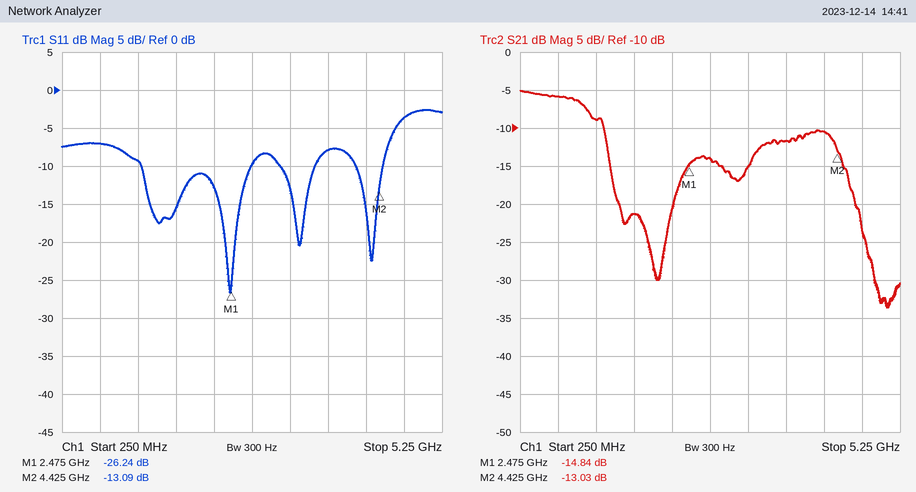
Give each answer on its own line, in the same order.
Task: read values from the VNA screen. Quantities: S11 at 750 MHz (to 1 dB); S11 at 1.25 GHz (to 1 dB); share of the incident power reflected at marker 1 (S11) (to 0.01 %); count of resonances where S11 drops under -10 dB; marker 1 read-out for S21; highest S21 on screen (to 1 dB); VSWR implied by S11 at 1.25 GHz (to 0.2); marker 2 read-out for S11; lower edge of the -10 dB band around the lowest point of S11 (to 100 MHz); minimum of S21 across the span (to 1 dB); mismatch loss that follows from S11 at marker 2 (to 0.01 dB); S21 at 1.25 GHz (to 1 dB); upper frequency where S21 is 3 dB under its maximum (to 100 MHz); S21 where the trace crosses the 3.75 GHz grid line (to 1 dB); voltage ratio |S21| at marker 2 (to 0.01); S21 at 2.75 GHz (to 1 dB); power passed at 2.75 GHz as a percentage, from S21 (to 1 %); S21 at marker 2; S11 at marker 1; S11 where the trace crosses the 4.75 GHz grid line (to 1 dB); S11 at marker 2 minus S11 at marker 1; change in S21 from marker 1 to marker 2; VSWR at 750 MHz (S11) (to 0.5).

-7 dB
-9 dB
0.24 %
4
-14.84 dB
-5 dB
2.0
-13.09 dB
1.3 GHz
-34 dB
0.22 dB
-9 dB
1.2 GHz
-12 dB
0.22
-14 dB
4 %
-13.03 dB
-26.24 dB
-4 dB
13.15 dB
1.81 dB
2.5
